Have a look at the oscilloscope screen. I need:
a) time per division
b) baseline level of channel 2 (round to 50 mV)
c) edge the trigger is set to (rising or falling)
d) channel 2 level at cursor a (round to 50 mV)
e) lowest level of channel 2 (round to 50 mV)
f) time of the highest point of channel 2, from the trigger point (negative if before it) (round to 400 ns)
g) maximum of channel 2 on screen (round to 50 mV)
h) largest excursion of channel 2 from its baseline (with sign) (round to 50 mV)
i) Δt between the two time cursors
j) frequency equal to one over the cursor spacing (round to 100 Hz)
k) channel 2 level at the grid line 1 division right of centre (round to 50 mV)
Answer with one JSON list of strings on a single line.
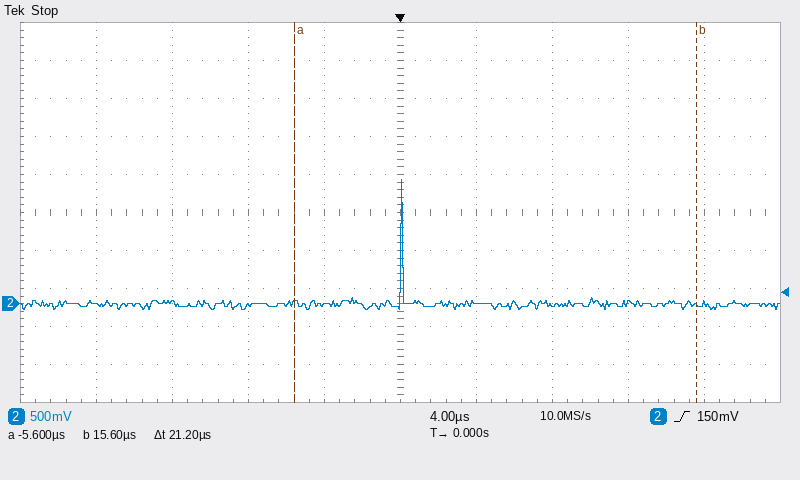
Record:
["4 µs", "0 mV", "rising", "0 mV", "-100 mV", "0.0 µs", "1.65 V", "+1.65 V", "21.2 µs", "47.2 kHz", "0 mV"]
